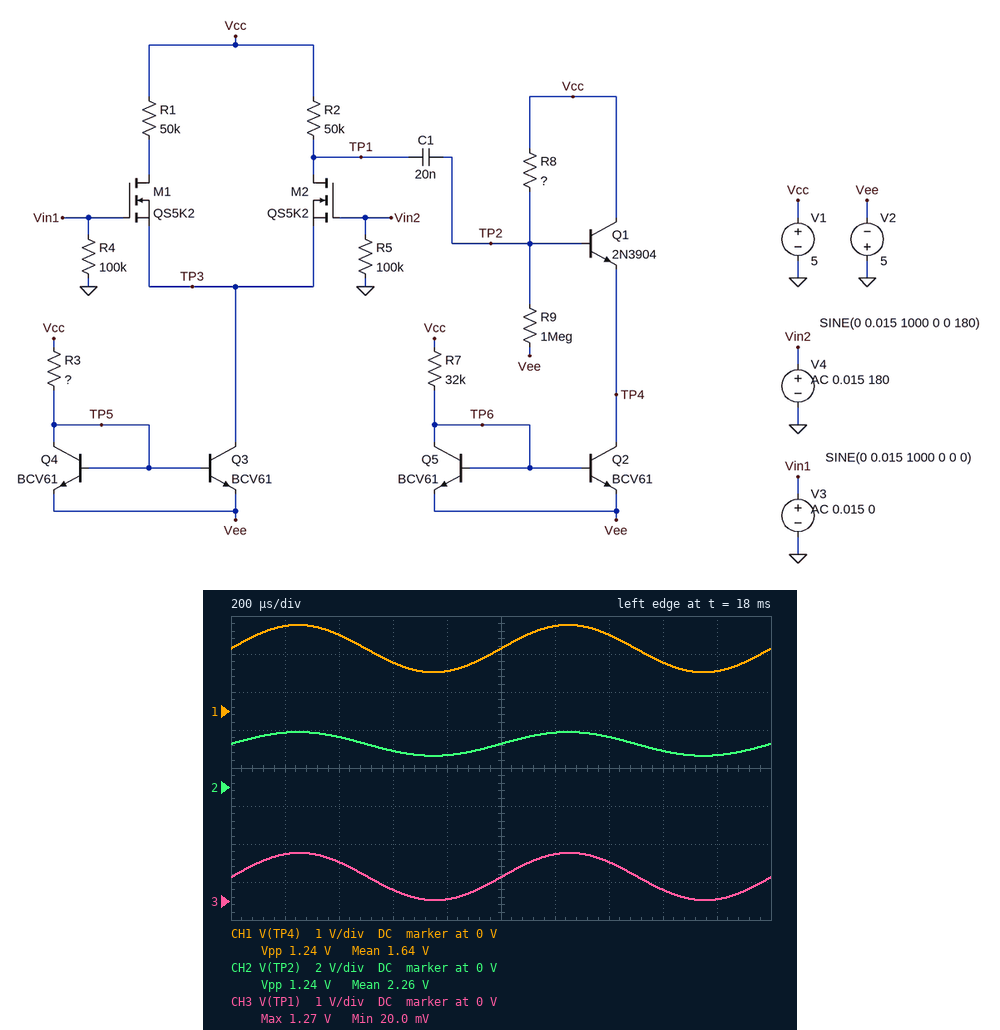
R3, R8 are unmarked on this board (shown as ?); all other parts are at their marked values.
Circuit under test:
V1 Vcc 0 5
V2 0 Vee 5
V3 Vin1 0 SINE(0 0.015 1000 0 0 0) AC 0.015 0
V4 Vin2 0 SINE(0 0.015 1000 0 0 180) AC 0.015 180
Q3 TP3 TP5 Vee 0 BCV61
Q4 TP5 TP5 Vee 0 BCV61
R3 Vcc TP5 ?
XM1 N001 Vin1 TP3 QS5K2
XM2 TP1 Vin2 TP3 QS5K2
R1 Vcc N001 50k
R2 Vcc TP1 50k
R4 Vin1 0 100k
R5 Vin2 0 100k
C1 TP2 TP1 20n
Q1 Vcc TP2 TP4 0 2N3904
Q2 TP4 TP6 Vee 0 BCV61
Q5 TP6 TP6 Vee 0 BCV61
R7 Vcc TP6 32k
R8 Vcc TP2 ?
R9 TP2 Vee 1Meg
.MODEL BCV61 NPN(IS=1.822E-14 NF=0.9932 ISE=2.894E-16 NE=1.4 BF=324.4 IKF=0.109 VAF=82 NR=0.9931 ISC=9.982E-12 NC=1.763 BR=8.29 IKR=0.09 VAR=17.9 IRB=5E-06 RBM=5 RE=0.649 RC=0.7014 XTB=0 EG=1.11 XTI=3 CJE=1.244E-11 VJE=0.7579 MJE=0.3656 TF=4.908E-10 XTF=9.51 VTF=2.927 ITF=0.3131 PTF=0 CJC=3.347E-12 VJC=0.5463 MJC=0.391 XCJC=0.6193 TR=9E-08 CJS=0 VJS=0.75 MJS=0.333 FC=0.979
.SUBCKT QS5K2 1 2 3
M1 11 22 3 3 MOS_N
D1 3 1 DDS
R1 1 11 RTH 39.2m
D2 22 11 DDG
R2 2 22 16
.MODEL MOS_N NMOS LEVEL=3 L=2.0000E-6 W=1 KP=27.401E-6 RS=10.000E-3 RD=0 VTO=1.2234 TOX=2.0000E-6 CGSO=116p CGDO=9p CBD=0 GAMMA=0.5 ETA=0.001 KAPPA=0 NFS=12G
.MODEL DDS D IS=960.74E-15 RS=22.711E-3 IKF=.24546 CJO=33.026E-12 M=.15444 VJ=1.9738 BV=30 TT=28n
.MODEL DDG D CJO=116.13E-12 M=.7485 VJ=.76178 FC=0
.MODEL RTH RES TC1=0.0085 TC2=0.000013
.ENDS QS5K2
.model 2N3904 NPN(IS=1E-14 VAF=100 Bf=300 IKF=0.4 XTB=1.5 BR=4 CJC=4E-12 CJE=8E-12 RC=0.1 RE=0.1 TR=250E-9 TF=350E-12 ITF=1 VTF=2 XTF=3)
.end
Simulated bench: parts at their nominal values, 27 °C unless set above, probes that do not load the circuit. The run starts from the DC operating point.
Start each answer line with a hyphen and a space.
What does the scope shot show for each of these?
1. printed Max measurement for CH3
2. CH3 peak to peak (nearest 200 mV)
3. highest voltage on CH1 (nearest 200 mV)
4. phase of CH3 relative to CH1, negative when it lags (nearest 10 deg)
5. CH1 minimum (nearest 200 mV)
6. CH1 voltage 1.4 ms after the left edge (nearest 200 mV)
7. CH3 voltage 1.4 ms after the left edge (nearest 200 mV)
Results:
- 1.27 V
- 1.2 V
- 2.2 V
- 0 deg
- 1.0 V
- 2.0 V
- 1.0 V
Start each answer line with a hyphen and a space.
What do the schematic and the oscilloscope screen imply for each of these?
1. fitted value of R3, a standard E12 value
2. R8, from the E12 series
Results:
- 56 kΩ
- 330 kΩ
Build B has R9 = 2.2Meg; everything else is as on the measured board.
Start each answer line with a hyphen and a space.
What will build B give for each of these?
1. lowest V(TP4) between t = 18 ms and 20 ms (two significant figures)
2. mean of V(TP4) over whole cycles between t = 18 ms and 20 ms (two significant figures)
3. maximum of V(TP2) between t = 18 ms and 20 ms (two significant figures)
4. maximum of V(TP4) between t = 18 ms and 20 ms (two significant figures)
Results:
- 2.1 V
- 2.8 V
- 4.0 V
- 3.4 V
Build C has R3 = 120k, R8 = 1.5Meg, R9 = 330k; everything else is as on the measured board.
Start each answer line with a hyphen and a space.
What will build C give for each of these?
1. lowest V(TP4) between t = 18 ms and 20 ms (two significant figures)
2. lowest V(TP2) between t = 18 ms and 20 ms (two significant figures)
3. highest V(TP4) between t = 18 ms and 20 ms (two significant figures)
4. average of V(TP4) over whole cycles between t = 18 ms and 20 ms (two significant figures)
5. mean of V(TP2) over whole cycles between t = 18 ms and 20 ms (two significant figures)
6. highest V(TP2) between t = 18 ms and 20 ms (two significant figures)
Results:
- -4.4 V
- -3.8 V
- -3.7 V
- -4.1 V
- -3.4 V
- -3.1 V
